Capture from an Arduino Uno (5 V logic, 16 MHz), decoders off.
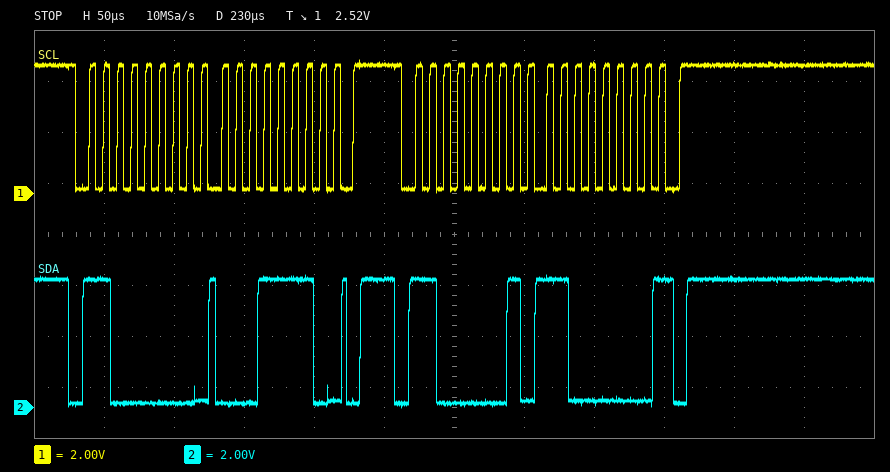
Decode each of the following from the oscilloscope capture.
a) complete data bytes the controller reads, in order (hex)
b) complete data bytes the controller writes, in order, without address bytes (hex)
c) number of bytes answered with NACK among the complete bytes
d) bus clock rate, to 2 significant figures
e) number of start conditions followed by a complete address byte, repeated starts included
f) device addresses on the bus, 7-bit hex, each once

C0
1E
1
100 kHz
2
0x60
